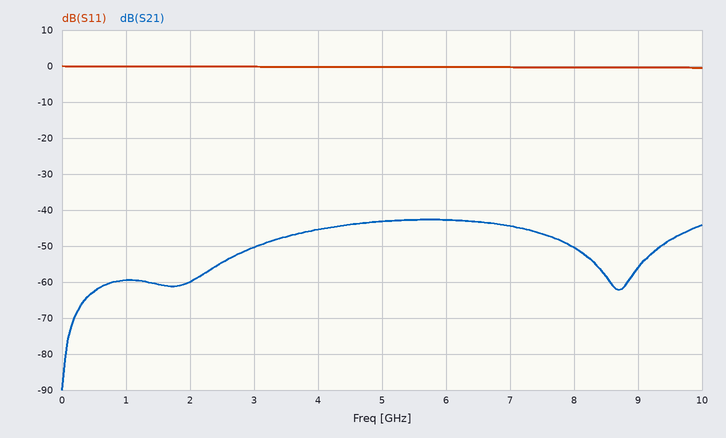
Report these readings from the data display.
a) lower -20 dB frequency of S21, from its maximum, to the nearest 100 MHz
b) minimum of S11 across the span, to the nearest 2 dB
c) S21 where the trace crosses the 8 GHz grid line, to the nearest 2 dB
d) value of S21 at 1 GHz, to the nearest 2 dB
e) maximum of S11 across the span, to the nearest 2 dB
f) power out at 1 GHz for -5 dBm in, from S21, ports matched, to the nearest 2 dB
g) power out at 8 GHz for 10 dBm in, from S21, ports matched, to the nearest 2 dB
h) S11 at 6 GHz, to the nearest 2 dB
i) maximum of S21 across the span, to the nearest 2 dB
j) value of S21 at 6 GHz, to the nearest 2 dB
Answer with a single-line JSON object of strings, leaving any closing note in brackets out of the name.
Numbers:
{"lower -20 dB frequency of S21, from its maximum, to the nearest 100 MHz": "500 MHz", "minimum of S11 across the span, to the nearest 2 dB": "0 dB", "S21 where the trace crosses the 8 GHz grid line, to the nearest 2 dB": "-50 dB", "value of S21 at 1 GHz, to the nearest 2 dB": "-60 dB", "maximum of S11 across the span, to the nearest 2 dB": "0 dB", "power out at 1 GHz for -5 dBm in, from S21, ports matched, to the nearest 2 dB": "-64 dBm", "power out at 8 GHz for 10 dBm in, from S21, ports matched, to the nearest 2 dB": "-40 dBm", "S11 at 6 GHz, to the nearest 2 dB": "0 dB", "maximum of S21 across the span, to the nearest 2 dB": "-42 dB", "value of S21 at 6 GHz, to the nearest 2 dB": "-42 dB"}
